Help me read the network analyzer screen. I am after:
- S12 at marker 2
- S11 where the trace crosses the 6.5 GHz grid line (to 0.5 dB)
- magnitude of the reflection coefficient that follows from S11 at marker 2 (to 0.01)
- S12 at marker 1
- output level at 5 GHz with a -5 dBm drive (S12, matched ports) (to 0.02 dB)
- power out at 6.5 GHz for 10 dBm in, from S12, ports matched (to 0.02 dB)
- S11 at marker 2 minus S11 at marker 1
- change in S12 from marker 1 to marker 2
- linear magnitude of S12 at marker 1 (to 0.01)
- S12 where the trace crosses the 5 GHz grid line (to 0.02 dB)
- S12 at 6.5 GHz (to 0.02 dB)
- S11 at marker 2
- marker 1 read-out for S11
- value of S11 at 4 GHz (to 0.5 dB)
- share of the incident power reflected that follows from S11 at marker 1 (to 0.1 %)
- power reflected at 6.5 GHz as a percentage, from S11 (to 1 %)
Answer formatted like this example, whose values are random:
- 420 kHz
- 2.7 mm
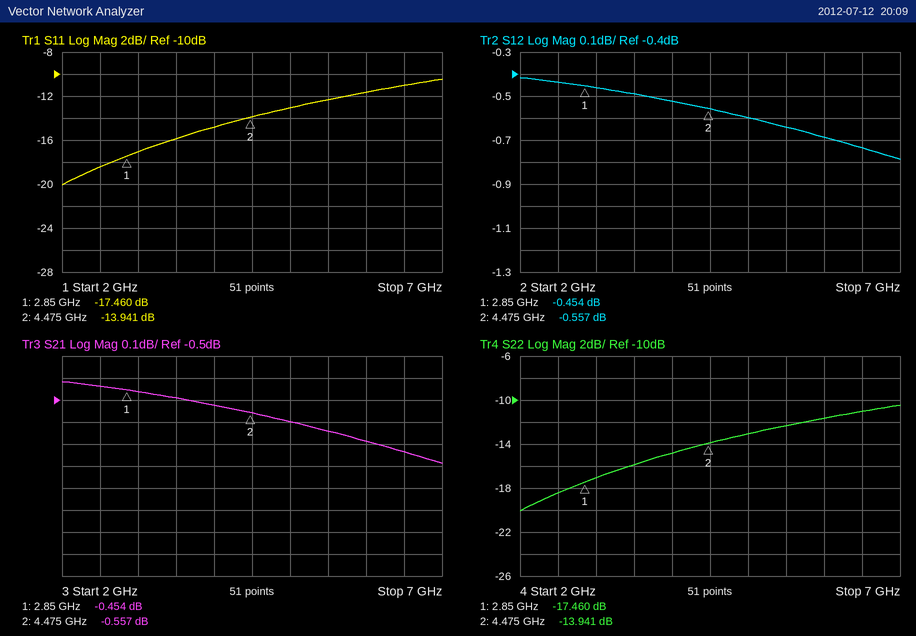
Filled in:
- -0.557 dB
- -11.0 dB
- 0.20
- -0.454 dB
- -5.60 dBm
- 9.26 dBm
- 3.519 dB
- -0.103 dB
- 0.95
- -0.60 dB
- -0.74 dB
- -13.941 dB
- -17.460 dB
- -15.0 dB
- 1.8 %
- 8 %
